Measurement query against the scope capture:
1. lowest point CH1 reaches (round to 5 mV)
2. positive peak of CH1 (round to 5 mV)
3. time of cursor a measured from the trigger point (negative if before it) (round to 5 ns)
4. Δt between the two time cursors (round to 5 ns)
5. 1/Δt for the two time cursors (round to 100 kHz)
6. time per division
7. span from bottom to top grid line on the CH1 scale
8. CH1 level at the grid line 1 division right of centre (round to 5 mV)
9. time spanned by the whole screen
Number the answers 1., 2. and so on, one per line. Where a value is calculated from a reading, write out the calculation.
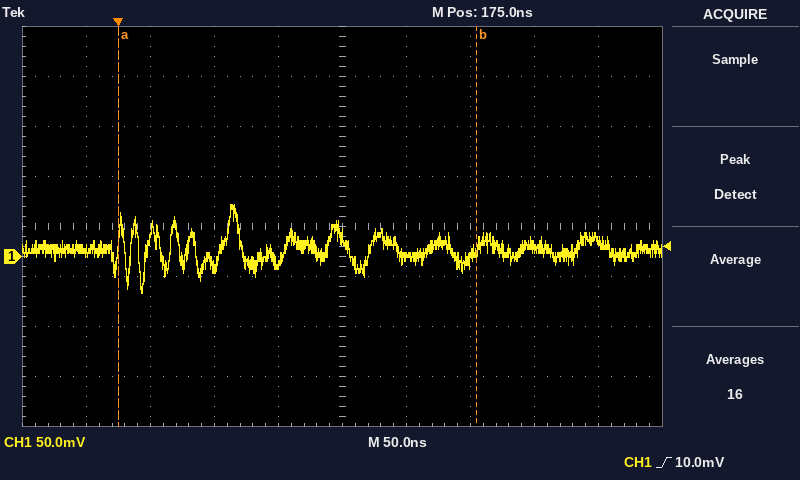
1. -35 mV
2. 50 mV
3. 0 ns
4. 280 ns
5. 1 / 280 ns ≈ 3.6 MHz
6. 50 ns
7. 400 mV
8. 0 mV
9. 500 ns
